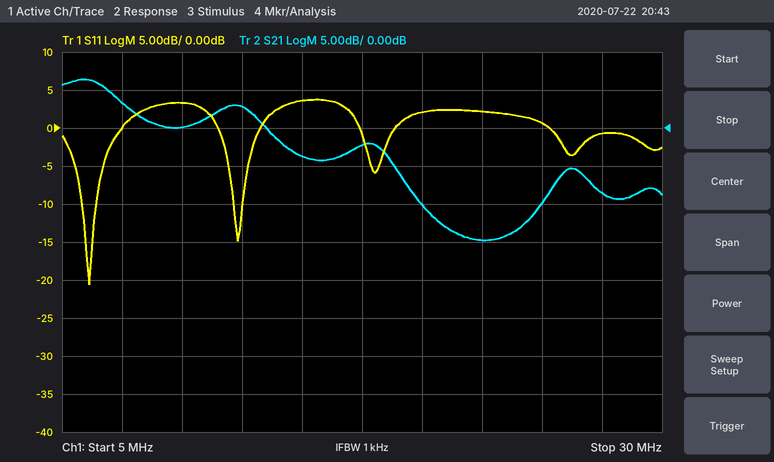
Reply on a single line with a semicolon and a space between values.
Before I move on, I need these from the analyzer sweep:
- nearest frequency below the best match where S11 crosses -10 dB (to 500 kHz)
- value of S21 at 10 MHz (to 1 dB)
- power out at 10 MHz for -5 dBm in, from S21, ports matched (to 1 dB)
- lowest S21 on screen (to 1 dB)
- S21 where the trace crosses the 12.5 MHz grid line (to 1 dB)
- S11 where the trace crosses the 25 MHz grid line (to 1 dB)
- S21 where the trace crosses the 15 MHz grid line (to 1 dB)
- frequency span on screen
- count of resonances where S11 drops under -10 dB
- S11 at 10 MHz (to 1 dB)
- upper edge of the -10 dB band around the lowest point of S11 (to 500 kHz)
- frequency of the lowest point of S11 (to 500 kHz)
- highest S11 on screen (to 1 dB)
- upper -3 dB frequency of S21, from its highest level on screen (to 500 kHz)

6.0 MHz; 0 dB; -5 dBm; -15 dB; 3 dB; 1 dB; -4 dB; 25 MHz; 2; 3 dB; 6.5 MHz; 6.0 MHz; 4 dB; 7.5 MHz
